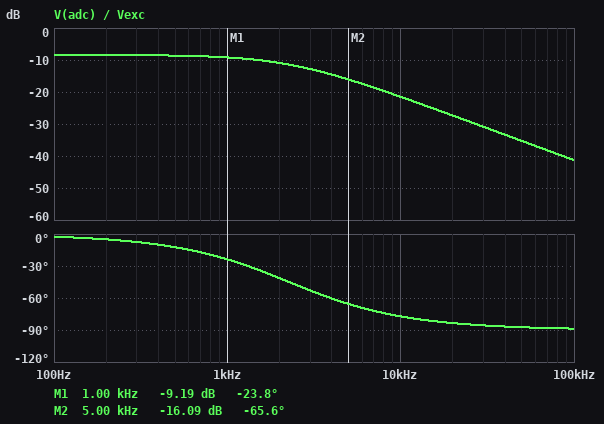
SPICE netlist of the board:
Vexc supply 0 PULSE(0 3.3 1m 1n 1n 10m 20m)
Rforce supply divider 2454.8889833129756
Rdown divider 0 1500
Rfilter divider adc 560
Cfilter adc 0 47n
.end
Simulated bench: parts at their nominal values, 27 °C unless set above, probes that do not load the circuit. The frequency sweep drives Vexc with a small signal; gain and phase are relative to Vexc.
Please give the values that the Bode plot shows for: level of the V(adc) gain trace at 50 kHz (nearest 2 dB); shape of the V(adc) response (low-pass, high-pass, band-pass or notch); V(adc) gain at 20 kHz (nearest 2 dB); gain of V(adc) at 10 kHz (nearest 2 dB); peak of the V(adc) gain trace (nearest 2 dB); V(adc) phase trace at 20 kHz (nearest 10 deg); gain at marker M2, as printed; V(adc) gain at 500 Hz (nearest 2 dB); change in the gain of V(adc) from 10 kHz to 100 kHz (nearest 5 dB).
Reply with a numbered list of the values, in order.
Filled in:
1. -36 dB
2. low-pass
3. -28 dB
4. -22 dB
5. -8 dB
6. -80 deg
7. -16.09 dB
8. -8 dB
9. -20 dB
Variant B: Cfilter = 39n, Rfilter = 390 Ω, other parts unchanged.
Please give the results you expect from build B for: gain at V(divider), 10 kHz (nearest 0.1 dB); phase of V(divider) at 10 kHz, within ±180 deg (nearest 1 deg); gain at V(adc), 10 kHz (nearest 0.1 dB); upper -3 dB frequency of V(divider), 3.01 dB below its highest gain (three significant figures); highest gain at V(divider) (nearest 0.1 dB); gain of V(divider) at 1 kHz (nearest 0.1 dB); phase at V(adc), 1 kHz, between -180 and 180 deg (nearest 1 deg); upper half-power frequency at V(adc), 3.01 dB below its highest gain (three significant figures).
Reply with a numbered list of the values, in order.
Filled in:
1. -16.2 dB
2. -29 deg
3. -19.0 dB
4. 3.40 kHz
5. -8.4 dB
6. -8.8 dB
7. -18 deg
8. 3.09 kHz
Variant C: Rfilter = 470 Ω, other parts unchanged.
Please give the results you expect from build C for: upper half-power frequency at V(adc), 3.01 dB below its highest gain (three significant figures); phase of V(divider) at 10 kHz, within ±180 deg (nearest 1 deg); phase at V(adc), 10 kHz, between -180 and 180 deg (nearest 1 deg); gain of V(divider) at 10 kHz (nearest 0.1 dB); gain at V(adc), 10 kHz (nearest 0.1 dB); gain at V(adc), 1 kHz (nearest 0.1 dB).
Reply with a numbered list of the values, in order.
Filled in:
1. 2.42 kHz
2. -22 deg
3. -76 deg
4. -16.3 dB
5. -21.0 dB
6. -9.1 dB
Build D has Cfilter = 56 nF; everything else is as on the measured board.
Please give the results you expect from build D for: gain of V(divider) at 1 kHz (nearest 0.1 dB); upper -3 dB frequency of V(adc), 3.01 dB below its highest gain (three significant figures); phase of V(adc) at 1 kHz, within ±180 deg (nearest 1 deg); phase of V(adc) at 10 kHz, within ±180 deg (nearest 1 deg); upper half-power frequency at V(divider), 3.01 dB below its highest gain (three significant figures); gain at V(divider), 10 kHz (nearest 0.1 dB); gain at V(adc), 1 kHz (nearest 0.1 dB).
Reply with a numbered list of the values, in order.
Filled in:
1. -9.3 dB
2. 1.91 kHz
3. -28 deg
4. -79 deg
5. 2.25 kHz
6. -16.1 dB
7. -9.5 dB
